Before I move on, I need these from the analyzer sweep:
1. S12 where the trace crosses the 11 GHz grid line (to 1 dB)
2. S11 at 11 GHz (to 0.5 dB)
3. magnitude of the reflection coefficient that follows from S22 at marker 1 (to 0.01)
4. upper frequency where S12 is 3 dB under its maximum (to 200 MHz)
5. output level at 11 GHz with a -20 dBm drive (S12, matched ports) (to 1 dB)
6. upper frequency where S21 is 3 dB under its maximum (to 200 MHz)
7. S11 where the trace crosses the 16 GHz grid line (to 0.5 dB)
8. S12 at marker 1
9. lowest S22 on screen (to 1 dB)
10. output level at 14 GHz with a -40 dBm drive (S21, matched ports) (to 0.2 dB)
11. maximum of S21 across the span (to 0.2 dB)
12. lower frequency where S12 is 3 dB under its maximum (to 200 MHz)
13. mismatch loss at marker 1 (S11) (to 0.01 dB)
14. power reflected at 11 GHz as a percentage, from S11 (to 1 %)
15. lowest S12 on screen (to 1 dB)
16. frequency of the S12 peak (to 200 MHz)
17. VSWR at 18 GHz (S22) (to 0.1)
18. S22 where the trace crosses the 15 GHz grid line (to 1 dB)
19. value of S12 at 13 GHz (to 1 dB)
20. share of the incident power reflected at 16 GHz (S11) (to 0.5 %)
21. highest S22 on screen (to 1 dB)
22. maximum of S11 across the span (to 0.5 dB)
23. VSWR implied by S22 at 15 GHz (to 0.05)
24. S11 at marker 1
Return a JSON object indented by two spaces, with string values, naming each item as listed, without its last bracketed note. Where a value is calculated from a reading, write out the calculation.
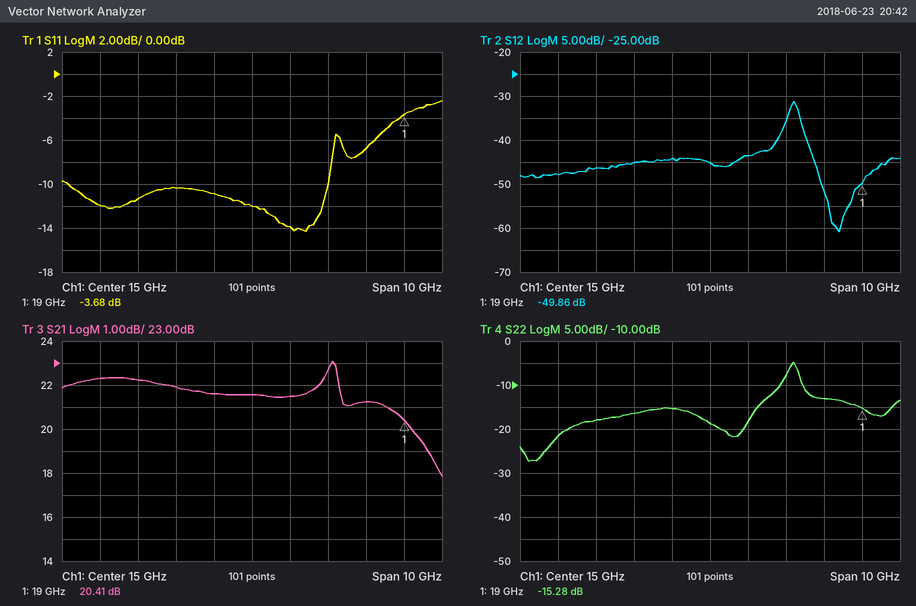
{
  "S12 where the trace crosses the 11 GHz grid line": "-48 dB",
  "S11 at 11 GHz": "-12.0 dB",
  "magnitude of the reflection coefficient that follows from S22 at marker 1": "10^(-15.28/20) ≈ 0.17",
  "upper frequency where S12 is 3 dB under its maximum": "17.4 GHz",
  "output level at 11 GHz with a -20 dBm drive (S12, matched ports)": "-20 dBm + (-48 dB) = -68 dBm",
  "upper frequency where S21 is 3 dB under its maximum": "19.2 GHz",
  "S11 where the trace crosses the 16 GHz grid line": "-14.0 dB",
  "S12 at marker 1": "-49.86 dB",
  "lowest S22 on screen": "-27 dB",
  "output level at 14 GHz with a -40 dBm drive (S21, matched ports)": "-40 dBm + (21.6 dB) = -18.4 dBm",
  "maximum of S21 across the span": "23.0 dB",
  "lower frequency where S12 is 3 dB under its maximum": "17.0 GHz",
  "mismatch loss at marker 1 (S11)": "−10 log10(1 − 10^(-3.68/10)) ≈ 2.43 dB",
  "power reflected at 11 GHz as a percentage, from S11": "10^(-12/10) ≈ 6 %",
  "lowest S12 on screen": "-61 dB",
  "frequency of the S12 peak": "17.2 GHz",
  "VSWR at 18 GHz (S22)": "|Γ| = 10^(-13/20) = 0.2239; VSWR = (1 + 0.2239)/(1 − 0.2239) ≈ 1.6",
  "S22 where the trace crosses the 15 GHz grid line": "-19 dB",
  "value of S12 at 13 GHz": "-45 dB",
  "share of the incident power reflected at 16 GHz (S11)": "10^(-14/10) ≈ 4.0 %",
  "highest S22 on screen": "-5 dB",
  "maximum of S11 across the span": "-2.5 dB",
  "VSWR implied by S22 at 15 GHz": "|Γ| = 10^(-19/20) = 0.1122; VSWR = (1 + 0.1122)/(1 − 0.1122) ≈ 1.25",
  "S11 at marker 1": "-3.68 dB"
}
